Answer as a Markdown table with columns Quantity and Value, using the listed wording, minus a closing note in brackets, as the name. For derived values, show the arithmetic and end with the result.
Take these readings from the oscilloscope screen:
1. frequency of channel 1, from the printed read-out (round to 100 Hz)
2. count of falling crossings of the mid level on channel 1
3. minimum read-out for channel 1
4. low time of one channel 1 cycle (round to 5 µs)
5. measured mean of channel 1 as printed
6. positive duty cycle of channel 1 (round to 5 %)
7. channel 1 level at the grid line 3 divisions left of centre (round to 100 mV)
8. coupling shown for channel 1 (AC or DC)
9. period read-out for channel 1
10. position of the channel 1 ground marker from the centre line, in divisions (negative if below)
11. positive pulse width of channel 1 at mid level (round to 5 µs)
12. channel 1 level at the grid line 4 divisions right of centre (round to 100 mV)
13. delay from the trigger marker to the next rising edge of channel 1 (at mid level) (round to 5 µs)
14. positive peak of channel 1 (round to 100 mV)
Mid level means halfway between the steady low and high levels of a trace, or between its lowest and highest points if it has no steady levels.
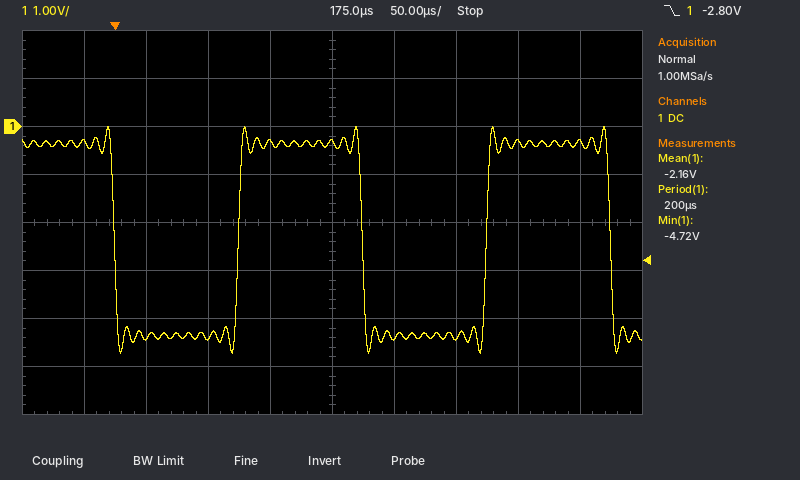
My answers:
| Quantity | Value |
|---|---|
| frequency of channel 1, from the printed read-out | 1 / 200 µs ≈ 5.0 kHz |
| count of falling crossings of the mid level on channel 1 | 3 |
| minimum read-out for channel 1 | -4.72 V |
| low time of one channel 1 cycle | 100 µs |
| measured mean of channel 1 as printed | -2.16 V |
| positive duty cycle of channel 1 | 50 % |
| channel 1 level at the grid line 3 divisions left of centre | -4.4 V |
| coupling shown for channel 1 | DC |
| period read-out for channel 1 | 200 µs |
| position of the channel 1 ground marker from the centre line, in divisions | +2.0 div |
| positive pulse width of channel 1 at mid level | 100 µs |
| channel 1 level at the grid line 4 divisions right of centre | -300 mV |
| delay from the trigger marker to the next rising edge of channel 1 (at mid level) | 100 µs |
| positive peak of channel 1 | 0.0 V |
